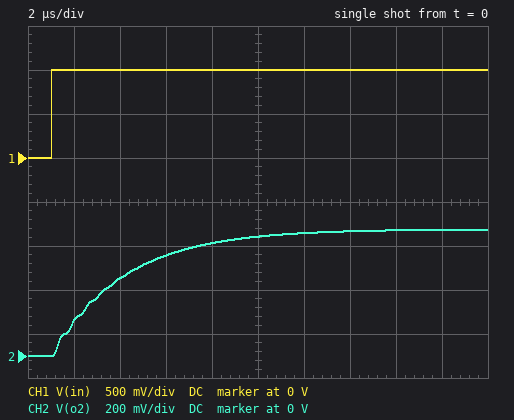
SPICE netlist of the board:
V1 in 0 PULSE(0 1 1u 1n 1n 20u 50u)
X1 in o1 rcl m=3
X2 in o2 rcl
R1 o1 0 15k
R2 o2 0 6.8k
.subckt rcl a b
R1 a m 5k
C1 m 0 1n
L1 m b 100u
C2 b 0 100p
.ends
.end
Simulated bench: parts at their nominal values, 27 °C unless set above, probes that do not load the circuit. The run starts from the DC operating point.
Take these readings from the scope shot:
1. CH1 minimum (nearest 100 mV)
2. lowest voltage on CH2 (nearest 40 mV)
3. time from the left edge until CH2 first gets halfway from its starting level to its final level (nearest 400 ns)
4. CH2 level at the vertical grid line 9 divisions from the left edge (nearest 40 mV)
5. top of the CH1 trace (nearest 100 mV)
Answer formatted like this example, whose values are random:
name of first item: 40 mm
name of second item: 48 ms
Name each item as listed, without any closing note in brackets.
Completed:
CH1 minimum: 0 V
lowest voltage on CH2: 0 V
time from the left edge until CH2 first gets halfway from its starting level to its final level: 3.2 µs
CH2 level at the vertical grid line 9 divisions from the left edge: 560 mV
top of the CH1 trace: 1.0 V
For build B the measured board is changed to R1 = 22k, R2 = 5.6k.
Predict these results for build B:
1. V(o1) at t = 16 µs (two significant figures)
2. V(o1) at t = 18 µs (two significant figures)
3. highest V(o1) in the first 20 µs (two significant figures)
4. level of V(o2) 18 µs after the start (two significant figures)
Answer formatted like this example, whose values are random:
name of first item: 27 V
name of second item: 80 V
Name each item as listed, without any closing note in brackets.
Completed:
V(o1) at t = 16 µs: 880 mV
V(o1) at t = 18 µs: 890 mV
highest V(o1) in the first 20 µs: 910 mV
level of V(o2) 18 µs after the start: 530 mV
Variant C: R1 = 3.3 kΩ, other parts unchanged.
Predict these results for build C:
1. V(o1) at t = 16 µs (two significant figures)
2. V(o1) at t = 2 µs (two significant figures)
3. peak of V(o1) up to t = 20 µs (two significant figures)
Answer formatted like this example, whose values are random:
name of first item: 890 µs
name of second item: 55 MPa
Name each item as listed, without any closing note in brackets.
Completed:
V(o1) at t = 16 µs: 650 mV
V(o1) at t = 2 µs: 170 mV
peak of V(o1) up to t = 20 µs: 660 mV
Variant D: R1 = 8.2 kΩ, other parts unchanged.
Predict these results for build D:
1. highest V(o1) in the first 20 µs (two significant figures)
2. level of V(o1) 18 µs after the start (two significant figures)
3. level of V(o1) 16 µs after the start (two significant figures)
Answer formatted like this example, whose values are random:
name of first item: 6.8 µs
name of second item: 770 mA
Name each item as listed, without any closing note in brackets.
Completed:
highest V(o1) in the first 20 µs: 820 mV
level of V(o1) 18 µs after the start: 810 mV
level of V(o1) 16 µs after the start: 800 mV
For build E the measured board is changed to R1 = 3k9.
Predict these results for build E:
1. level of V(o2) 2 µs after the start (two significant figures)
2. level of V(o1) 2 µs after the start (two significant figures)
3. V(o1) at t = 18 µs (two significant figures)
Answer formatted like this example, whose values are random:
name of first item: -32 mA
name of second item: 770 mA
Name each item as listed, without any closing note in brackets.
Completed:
level of V(o2) 2 µs after the start: 160 mV
level of V(o1) 2 µs after the start: 170 mV
V(o1) at t = 18 µs: 690 mV
